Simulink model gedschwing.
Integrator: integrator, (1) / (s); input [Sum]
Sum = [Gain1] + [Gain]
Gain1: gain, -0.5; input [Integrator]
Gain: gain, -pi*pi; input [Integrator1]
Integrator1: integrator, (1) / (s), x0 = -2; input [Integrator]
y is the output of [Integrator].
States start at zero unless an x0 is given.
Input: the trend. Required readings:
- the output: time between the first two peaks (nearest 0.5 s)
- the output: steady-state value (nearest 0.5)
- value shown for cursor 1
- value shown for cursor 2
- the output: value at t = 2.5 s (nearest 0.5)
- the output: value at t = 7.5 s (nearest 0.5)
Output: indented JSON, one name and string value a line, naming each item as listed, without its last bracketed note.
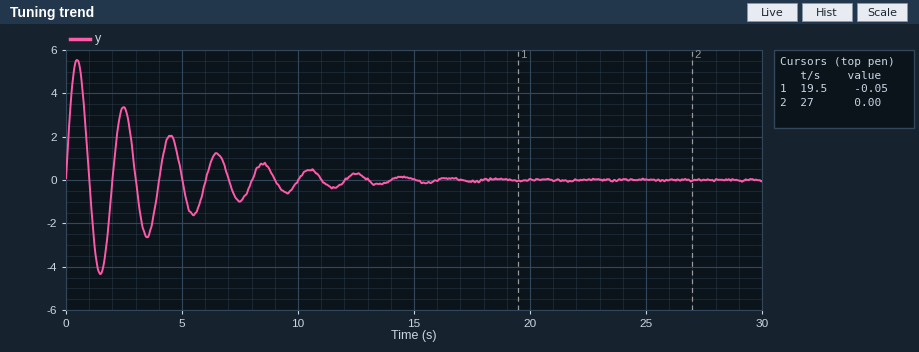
{
  "the output: time between the first two peaks": "2.0 s",
  "the output: steady-state value": "0.0",
  "value shown for cursor 1": "-0.05",
  "value shown for cursor 2": "0.00",
  "the output: value at t = 2.5 s": "3.5",
  "the output: value at t = 7.5 s": "-1.0"
}
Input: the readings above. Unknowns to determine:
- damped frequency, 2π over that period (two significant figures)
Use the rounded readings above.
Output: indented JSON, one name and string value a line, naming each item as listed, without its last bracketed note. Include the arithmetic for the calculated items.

{
  "damped frequency, 2π over that period": "2π / 2 = 3.1 rad/s"
}
